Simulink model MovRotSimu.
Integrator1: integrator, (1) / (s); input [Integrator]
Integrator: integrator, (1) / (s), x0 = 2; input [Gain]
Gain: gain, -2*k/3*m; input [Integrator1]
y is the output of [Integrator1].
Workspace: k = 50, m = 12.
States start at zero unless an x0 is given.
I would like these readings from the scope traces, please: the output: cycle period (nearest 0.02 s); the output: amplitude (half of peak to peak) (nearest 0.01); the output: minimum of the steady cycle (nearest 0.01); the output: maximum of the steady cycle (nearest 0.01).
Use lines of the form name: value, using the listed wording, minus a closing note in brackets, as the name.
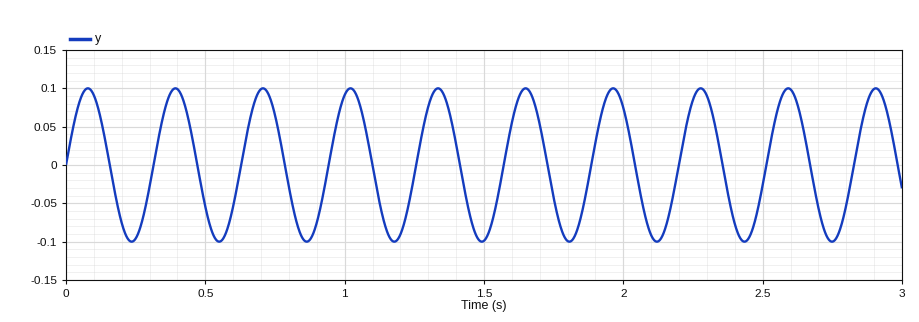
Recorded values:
the output: cycle period: 0.32 s
the output: amplitude (half of peak to peak): 0.10
the output: minimum of the steady cycle: -0.10
the output: maximum of the steady cycle: 0.10
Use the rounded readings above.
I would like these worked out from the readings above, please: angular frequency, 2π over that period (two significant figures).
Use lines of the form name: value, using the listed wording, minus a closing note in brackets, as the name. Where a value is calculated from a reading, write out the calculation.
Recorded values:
angular frequency, 2π over that period: 2π / 0.32 = 20 rad/s
